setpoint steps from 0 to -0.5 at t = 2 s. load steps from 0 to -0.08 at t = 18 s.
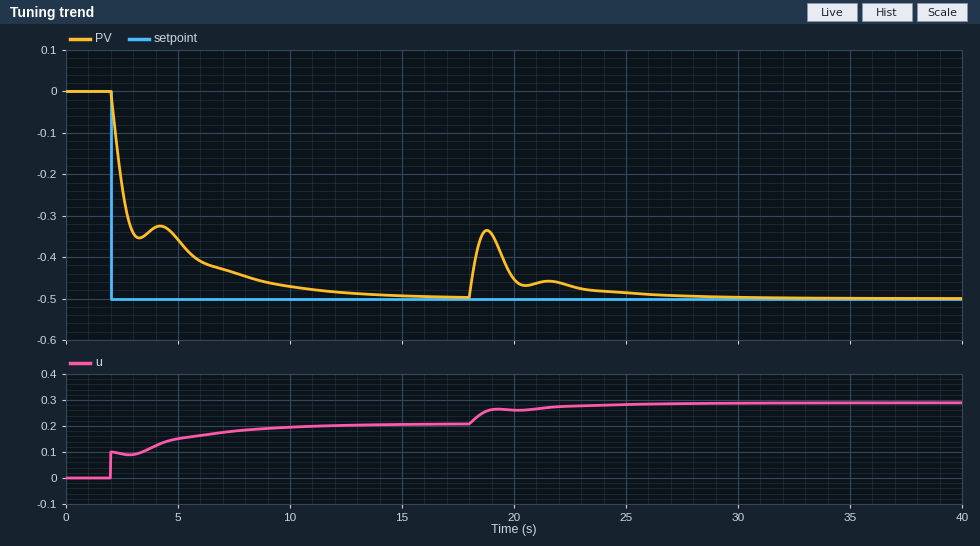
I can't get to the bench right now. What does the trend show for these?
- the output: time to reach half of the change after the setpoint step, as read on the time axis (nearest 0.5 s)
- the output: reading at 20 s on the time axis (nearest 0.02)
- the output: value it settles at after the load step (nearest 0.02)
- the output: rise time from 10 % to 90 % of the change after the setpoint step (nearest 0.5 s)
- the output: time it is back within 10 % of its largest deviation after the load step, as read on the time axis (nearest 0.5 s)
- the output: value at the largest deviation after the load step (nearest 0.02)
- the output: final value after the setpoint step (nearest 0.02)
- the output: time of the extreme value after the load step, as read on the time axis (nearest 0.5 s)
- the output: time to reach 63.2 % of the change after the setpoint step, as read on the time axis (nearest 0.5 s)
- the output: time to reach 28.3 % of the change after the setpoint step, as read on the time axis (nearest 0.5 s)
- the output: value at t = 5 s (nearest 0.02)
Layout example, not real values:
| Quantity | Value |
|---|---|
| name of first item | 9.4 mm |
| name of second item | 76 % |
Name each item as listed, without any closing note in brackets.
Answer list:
| Quantity | Value |
|---|---|
| the output: time to reach half of the change after the setpoint step, as read on the time axis | 2.5 s |
| the output: reading at 20 s on the time axis | -0.46 |
| the output: value it settles at after the load step | -0.50 |
| the output: rise time from 10 % to 90 % of the change after the setpoint step | 6.0 s |
| the output: time it is back within 10 % of its largest deviation after the load step, as read on the time axis | 24.5 s |
| the output: value at the largest deviation after the load step | -0.34 |
| the output: final value after the setpoint step | -0.50 |
| the output: time of the extreme value after the load step, as read on the time axis | 19.0 s |
| the output: time to reach 63.2 % of the change after the setpoint step, as read on the time axis | 3.0 s |
| the output: time to reach 28.3 % of the change after the setpoint step, as read on the time axis | 2.5 s |
| the output: value at t = 5 s | -0.36 |
